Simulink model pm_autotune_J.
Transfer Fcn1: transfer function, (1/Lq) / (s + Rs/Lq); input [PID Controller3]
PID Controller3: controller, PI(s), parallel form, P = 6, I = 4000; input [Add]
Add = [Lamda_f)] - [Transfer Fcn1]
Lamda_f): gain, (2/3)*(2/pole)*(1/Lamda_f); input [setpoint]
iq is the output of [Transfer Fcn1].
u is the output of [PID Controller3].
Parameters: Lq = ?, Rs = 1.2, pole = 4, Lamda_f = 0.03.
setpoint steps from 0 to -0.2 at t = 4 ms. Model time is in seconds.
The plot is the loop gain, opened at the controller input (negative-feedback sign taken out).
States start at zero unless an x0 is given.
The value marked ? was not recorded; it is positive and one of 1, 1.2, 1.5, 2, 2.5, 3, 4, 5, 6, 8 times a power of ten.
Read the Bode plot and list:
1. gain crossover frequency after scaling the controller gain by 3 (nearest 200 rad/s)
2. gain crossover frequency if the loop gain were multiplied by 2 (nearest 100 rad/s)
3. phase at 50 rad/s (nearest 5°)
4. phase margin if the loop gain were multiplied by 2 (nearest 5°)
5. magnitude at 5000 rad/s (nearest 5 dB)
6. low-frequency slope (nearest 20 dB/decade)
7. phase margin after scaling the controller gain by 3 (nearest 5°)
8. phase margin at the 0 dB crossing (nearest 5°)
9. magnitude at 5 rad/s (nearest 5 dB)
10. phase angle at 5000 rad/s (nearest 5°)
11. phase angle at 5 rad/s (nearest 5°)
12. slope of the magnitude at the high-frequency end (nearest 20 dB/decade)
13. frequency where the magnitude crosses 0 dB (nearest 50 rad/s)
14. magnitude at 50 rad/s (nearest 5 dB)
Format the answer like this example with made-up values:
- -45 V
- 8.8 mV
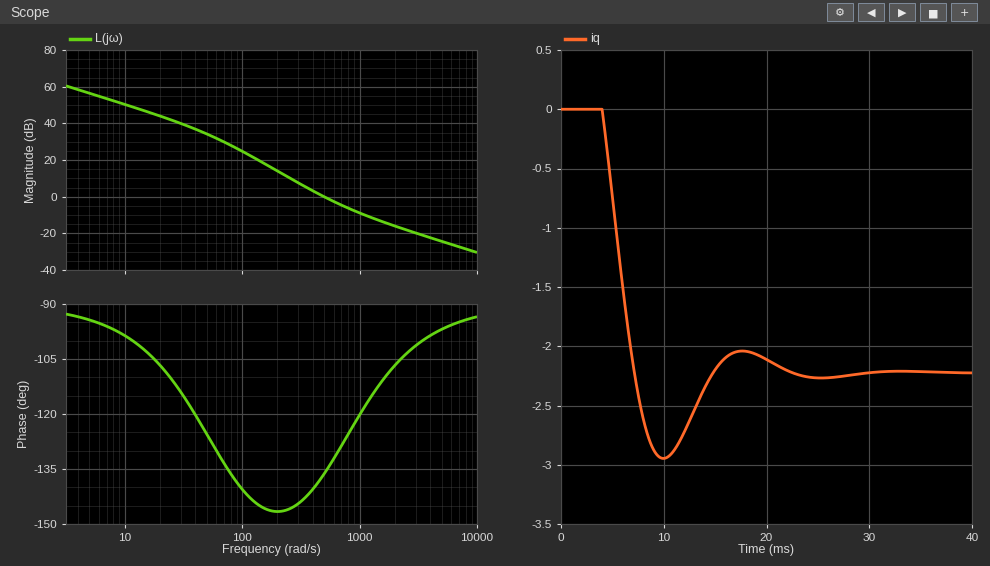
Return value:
- 1000 rad/s
- 800 rad/s
- -125°
- 55°
- -25 dB
- -20 dB/decade
- 60°
- 45°
- 55 dB
- -95°
- -95°
- -20 dB/decade
- 500 rad/s
- 35 dB
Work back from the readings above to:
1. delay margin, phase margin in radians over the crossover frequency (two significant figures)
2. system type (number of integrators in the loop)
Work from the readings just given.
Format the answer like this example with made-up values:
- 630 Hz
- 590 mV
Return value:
- 0.0016 s
- 1
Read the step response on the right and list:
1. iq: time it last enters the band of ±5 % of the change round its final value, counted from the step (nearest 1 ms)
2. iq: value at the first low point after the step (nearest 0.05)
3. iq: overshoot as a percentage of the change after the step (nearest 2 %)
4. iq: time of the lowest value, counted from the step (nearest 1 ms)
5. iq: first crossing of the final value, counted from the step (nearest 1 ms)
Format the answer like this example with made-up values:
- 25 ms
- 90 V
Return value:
- 16 ms
- -2.95
- 32 %
- 6 ms
- 3 ms
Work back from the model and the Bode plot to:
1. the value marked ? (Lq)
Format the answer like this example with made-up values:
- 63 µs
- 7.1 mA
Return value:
- 0.02
